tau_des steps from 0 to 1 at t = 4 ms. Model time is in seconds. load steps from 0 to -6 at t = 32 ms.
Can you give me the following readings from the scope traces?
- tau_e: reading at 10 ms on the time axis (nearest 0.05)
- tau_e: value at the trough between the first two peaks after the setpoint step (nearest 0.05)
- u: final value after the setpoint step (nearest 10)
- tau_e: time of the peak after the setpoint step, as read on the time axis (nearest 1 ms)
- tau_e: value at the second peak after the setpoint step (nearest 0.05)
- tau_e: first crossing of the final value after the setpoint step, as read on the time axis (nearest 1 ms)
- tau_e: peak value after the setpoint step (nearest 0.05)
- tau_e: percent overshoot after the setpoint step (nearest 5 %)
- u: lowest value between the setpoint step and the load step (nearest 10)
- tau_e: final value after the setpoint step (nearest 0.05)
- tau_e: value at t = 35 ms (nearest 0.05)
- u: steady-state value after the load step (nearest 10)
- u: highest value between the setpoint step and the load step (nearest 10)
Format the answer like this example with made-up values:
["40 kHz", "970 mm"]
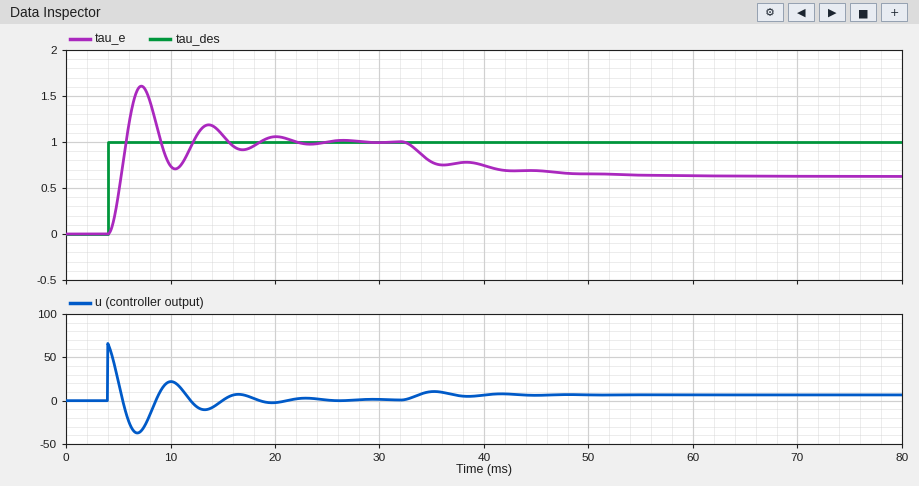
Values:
["0.75", "0.70", "0", "7 ms", "1.20", "6 ms", "1.60", "60 %", "-40", "1.00", "0.80", "10", "70"]
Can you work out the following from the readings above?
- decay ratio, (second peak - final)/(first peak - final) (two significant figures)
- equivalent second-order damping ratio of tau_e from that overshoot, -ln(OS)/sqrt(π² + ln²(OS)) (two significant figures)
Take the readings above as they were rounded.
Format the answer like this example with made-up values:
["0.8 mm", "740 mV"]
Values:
["0.33", "0.16"]
